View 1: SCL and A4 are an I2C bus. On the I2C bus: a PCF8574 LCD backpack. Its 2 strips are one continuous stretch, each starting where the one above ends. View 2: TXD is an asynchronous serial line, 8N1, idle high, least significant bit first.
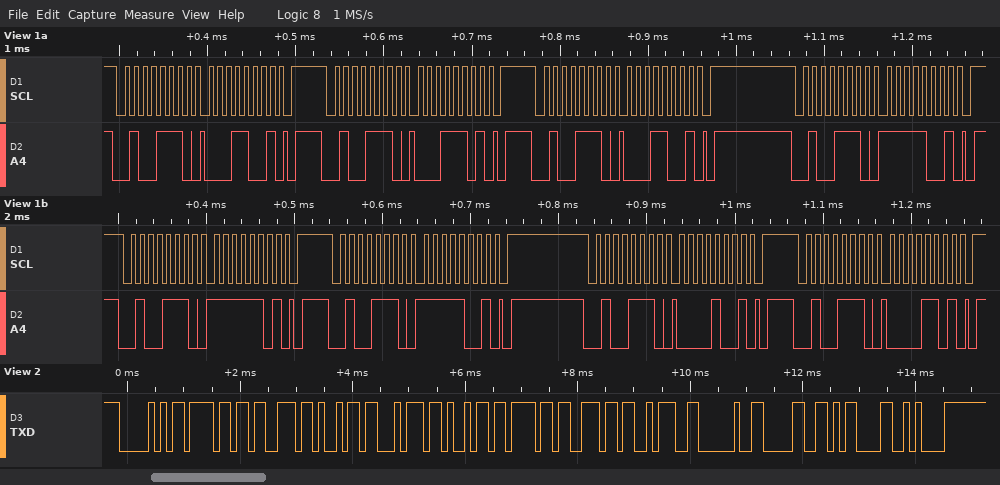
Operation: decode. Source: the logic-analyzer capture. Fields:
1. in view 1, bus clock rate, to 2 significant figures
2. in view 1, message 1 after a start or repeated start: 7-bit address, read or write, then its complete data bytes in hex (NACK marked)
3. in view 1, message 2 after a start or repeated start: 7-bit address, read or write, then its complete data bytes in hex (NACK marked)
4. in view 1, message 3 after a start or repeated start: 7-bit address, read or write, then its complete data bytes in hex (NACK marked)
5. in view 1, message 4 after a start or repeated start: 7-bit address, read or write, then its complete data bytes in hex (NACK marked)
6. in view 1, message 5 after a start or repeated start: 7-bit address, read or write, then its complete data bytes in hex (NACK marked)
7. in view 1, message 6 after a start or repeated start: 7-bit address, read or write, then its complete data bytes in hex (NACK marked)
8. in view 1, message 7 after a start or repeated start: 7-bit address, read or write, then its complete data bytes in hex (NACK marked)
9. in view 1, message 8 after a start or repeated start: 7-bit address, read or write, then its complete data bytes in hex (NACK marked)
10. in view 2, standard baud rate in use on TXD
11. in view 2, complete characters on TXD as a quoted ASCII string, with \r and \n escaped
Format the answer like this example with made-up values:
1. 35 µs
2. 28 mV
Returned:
1. 100 kHz
2. 0x27 write: 19
3. 0x27 write: 1D
4. 0x27 write: 19
5. 0x27 write: F9
6. 0x27 write: FD
7. 0x27 write: F9
8. 0x27 write: 09
9. 0x27 write: 0D
10. 9600 baud
11. "Position: 0\r\n"
